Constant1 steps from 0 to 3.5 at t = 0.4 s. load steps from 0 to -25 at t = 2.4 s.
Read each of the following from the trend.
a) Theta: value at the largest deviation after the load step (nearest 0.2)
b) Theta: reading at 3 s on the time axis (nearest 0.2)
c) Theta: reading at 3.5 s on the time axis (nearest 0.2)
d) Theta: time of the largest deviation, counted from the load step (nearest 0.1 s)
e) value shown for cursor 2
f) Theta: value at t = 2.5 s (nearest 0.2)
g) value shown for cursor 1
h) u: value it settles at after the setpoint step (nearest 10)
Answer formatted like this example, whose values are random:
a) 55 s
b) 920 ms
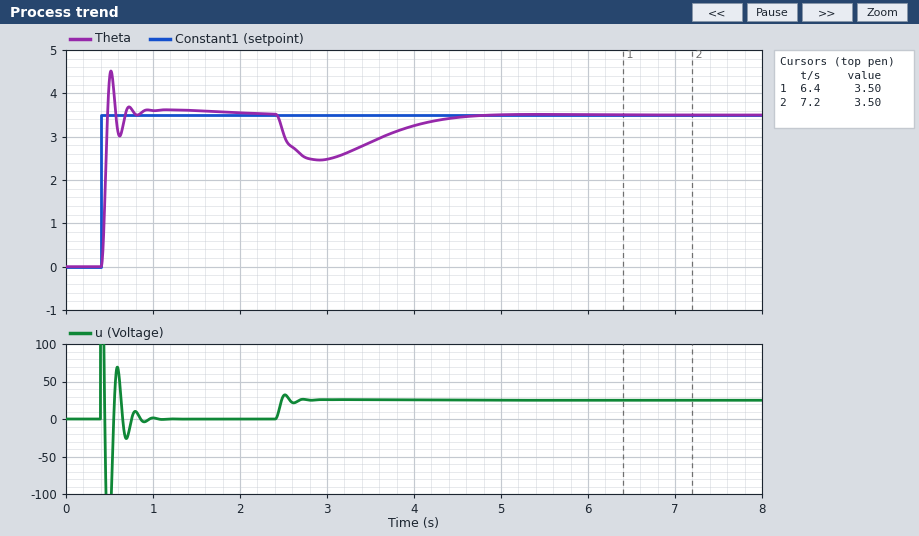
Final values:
a) 2.4
b) 2.4
c) 2.8
d) 0.5 s
e) 3.50
f) 3.0
g) 3.50
h) 0
